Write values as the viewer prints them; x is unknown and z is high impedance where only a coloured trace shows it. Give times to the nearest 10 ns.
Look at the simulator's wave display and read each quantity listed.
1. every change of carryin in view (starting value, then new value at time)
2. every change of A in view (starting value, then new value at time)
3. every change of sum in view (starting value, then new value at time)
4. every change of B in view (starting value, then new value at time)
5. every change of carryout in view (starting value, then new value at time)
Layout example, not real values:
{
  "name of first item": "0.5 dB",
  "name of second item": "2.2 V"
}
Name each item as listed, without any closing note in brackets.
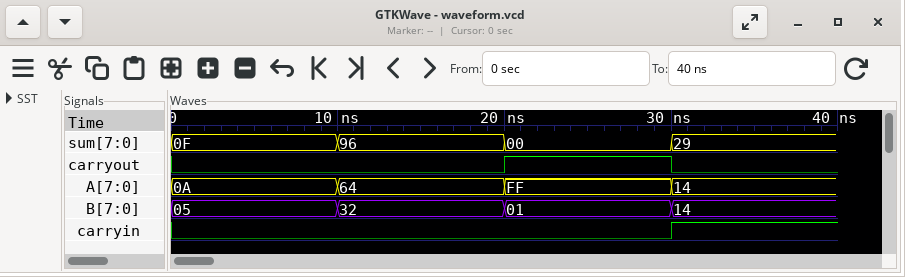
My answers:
{
  "every change of carryin in view": "0, 1 at 30 ns",
  "every change of A in view": "0A, 64 at 10 ns, FF at 20 ns, 14 at 30 ns",
  "every change of sum in view": "0F, 96 at 10 ns, 00 at 20 ns, 29 at 30 ns",
  "every change of B in view": "05, 32 at 10 ns, 01 at 20 ns, 14 at 30 ns",
  "every change of carryout in view": "0, 1 at 20 ns, 0 at 30 ns"
}
